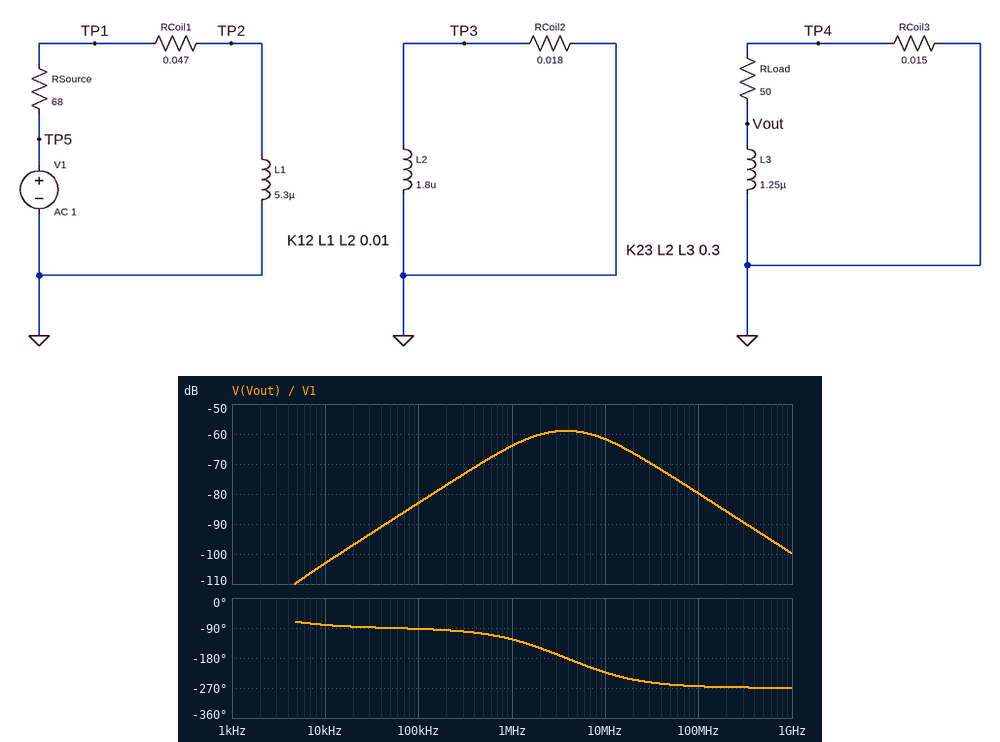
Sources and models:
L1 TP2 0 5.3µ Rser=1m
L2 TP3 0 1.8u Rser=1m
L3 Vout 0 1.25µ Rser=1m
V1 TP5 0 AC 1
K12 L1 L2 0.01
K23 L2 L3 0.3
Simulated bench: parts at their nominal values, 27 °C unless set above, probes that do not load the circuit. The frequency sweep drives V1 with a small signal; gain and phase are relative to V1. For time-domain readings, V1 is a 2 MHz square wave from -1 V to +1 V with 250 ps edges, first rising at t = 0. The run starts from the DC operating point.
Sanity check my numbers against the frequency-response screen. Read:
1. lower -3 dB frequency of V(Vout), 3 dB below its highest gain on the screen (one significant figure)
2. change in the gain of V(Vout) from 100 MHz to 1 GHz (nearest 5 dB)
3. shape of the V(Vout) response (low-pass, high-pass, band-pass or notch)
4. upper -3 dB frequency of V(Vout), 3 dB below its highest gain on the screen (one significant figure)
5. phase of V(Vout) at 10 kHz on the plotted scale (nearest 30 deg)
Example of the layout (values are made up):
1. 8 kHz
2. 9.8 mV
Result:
1. 1 MHz
2. -20 dB
3. band-pass
4. 10 MHz
5. -90 deg
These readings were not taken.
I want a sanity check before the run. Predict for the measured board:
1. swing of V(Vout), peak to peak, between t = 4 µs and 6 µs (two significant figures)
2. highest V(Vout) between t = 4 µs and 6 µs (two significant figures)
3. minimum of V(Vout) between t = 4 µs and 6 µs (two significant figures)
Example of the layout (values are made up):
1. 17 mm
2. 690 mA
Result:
1. 3.3 mV
2. 1.7 mV
3. -1.7 mV
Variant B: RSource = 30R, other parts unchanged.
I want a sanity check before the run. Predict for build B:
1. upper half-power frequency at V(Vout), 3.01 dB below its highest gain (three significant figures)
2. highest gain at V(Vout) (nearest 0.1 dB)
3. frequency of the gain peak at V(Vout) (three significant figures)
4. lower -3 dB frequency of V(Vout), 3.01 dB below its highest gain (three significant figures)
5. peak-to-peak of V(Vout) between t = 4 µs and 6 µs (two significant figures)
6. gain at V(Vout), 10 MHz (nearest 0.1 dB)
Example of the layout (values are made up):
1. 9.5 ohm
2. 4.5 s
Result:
1. 8.63 MHz
2. -57.8 dB
3. 2.51 MHz
4. 732 kHz
5. 3.4 mV
6. -61.6 dB
